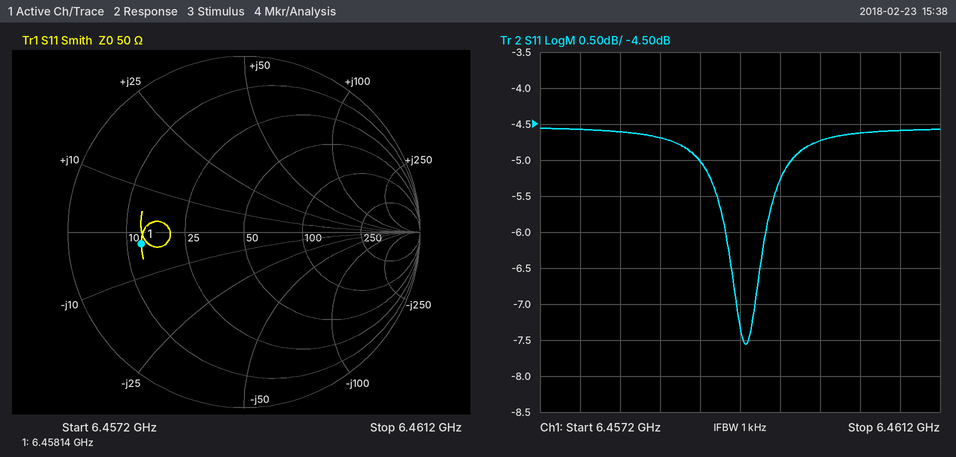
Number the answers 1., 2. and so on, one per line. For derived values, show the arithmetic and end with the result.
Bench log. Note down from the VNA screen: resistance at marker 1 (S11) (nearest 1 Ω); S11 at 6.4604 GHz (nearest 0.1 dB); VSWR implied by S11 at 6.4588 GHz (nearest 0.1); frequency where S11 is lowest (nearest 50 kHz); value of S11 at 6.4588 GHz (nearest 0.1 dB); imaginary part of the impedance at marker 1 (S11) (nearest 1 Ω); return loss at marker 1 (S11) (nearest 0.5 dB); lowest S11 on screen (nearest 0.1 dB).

1. 13 Ω
2. -4.6 dB
3. |Γ| = 10^(-5/20) = 0.5623; VSWR = (1 + 0.5623)/(1 − 0.5623) ≈ 3.6
4. 6.45925 GHz
5. -5.0 dB
6. -3 Ω
7. 4.5 dB
8. -7.6 dB
